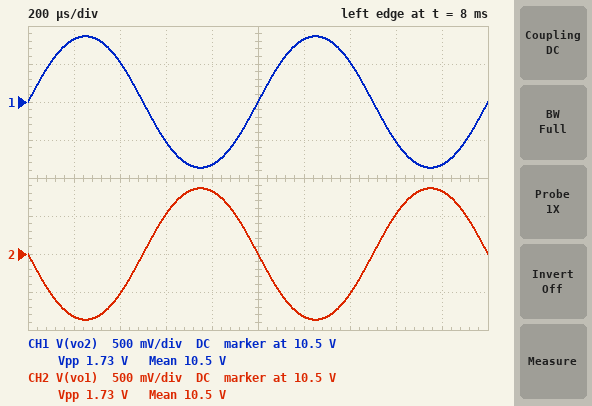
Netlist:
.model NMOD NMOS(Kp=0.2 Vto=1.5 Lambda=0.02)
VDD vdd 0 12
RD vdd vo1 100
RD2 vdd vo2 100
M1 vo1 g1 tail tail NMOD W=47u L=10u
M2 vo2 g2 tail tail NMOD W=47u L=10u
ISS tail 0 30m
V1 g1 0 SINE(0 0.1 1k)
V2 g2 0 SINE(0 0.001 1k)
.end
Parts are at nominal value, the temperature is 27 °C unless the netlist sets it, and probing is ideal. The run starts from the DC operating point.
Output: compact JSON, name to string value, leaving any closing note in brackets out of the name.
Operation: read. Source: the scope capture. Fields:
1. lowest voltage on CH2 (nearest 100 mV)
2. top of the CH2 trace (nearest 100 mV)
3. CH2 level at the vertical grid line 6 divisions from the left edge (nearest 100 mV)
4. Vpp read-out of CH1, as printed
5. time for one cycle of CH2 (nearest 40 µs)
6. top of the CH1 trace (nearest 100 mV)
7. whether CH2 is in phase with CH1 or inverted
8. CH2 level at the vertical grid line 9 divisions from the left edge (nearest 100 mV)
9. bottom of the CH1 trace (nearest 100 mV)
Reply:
{"lowest voltage on CH2": "9.6 V", "top of the CH2 trace": "11.4 V", "CH2 level at the vertical grid line 6 divisions from the left edge": "9.7 V", "Vpp read-out of CH1, as printed": "1.73 V", "time for one cycle of CH2": "1.00 ms", "top of the CH1 trace": "11.4 V", "whether CH2 is in phase with CH1 or inverted": "inverted", "CH2 level at the vertical grid line 9 divisions from the left edge": "11.3 V", "bottom of the CH1 trace": "9.6 V"}
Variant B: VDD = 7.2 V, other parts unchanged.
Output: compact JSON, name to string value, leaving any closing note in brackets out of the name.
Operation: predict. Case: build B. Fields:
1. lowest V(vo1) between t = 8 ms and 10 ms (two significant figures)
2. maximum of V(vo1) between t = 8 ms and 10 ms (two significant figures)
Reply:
{"lowest V(vo1) between t = 8 ms and 10 ms": "4.9 V", "maximum of V(vo1) between t = 8 ms and 10 ms": "6.5 V"}
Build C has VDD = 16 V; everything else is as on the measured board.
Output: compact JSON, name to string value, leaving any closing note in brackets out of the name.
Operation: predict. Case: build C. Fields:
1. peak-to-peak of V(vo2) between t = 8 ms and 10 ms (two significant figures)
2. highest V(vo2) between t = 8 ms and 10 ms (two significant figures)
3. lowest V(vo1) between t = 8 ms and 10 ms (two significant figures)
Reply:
{"peak-to-peak of V(vo2) between t = 8 ms and 10 ms": "1.8 V", "highest V(vo2) between t = 8 ms and 10 ms": "15 V", "lowest V(vo1) between t = 8 ms and 10 ms": "14 V"}
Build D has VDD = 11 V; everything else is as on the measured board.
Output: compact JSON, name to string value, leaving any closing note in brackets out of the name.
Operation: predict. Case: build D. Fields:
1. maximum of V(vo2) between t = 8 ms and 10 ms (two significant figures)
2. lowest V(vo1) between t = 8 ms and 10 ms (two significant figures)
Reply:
{"maximum of V(vo2) between t = 8 ms and 10 ms": "10 V", "lowest V(vo1) between t = 8 ms and 10 ms": "8.6 V"}
